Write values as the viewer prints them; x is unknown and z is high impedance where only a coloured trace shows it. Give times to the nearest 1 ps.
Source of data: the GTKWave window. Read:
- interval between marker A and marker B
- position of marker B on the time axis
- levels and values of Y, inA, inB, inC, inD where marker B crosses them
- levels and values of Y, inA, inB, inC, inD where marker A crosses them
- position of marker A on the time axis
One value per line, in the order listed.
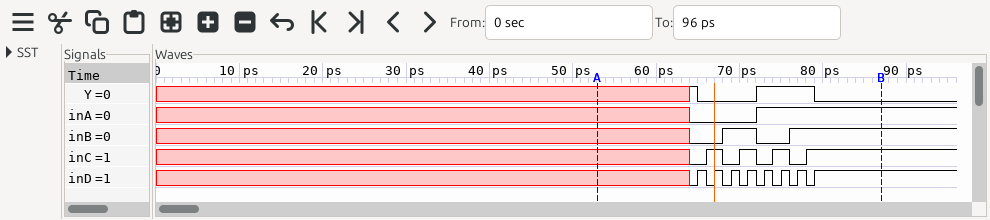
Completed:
34 ps
87 ps
Y=0, inA=1, inB=1, inC=1, inD=1
Y=x, inA=x, inB=x, inC=x, inD=x
53 ps
